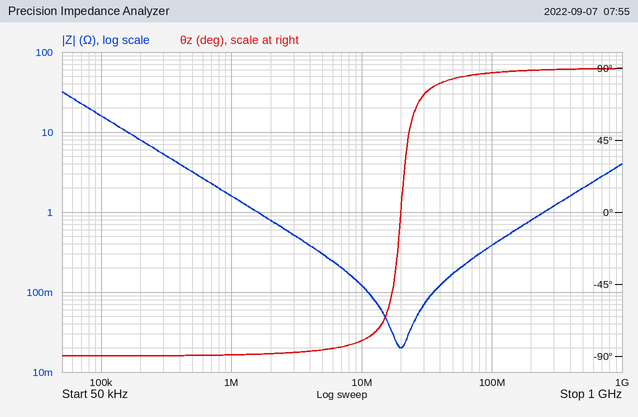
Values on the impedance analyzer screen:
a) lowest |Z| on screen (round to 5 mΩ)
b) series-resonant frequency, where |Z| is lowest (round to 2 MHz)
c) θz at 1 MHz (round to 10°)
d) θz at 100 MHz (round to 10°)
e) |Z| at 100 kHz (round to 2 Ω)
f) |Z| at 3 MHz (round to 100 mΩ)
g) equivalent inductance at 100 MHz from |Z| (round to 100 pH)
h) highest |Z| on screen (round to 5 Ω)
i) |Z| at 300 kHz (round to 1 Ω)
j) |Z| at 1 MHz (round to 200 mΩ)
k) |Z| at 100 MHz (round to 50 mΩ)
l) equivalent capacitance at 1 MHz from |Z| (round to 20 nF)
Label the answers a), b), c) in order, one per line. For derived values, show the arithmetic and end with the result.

a) 20 mΩ
b) 20 MHz
c) -90°
d) 90°
e) 16 Ω
f) 500 mΩ
g) L = 400 mΩ/(2π × 100 MHz) ≈ 637 pH, so 600 pH to the nearest 100 pH
h) 30 Ω
i) 5 Ω
j) 1.6 Ω
k) 400 mΩ
l) C = 1/(2π × 1 MHz × 1.6 Ω) ≈ 100 nF
